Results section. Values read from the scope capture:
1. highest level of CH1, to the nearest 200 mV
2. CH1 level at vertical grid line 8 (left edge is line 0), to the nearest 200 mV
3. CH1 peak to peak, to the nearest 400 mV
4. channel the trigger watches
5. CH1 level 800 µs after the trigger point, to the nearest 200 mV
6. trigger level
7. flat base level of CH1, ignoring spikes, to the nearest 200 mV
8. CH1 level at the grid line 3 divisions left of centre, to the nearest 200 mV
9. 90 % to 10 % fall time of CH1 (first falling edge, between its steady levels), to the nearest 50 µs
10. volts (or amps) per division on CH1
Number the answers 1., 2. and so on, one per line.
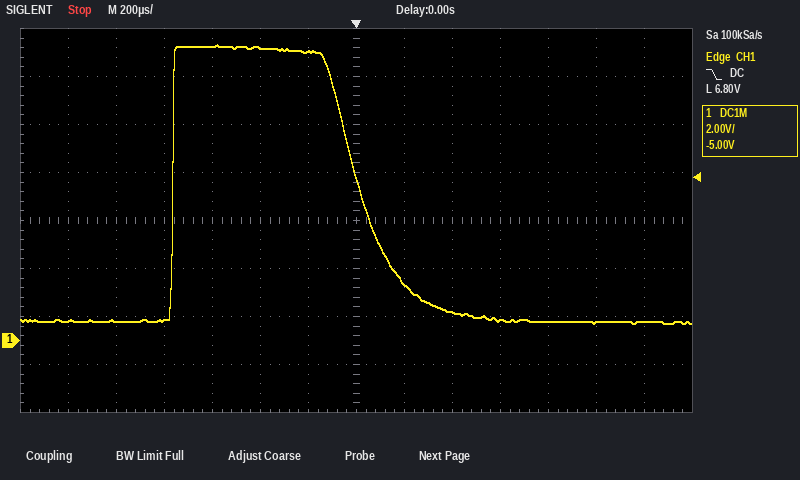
1. 12.4 V
2. 2.4 V
3. 11.6 V
4. CH1
5. 800 mV
6. 6.80 V
7. 800 mV
8. 12.2 V
9. 350 µs
10. 2 V
